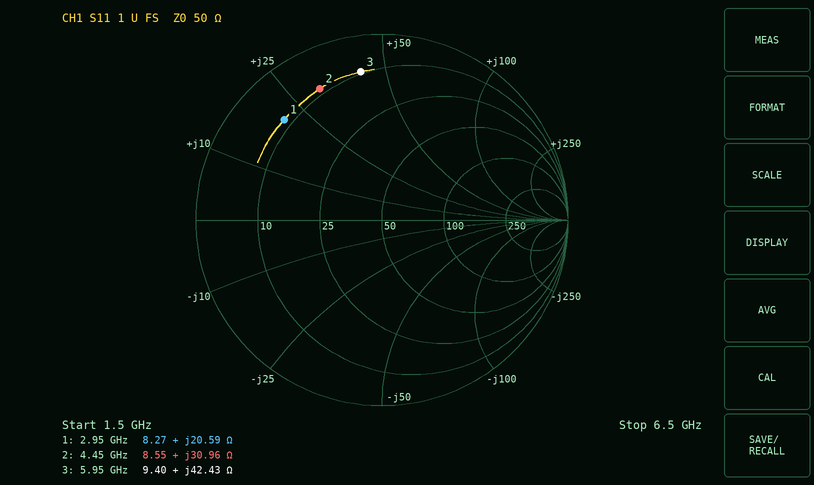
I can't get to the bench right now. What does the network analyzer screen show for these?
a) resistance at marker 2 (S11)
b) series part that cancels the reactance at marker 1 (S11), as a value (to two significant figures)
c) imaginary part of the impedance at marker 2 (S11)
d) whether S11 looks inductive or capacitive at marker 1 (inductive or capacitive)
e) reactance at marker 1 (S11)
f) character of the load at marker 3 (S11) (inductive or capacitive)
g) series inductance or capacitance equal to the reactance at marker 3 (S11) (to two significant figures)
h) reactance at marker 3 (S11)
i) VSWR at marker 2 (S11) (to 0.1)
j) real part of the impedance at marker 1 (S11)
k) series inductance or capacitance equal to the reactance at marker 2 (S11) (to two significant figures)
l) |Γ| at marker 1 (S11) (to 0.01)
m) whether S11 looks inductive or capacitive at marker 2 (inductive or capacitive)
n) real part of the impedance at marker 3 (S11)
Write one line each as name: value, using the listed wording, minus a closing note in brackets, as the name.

resistance at marker 2: 8.55 Ω
series part that cancels the reactance at marker 1 (S11), as a value: 2.6 pF
imaginary part of the impedance at marker 2: +30.96 Ω
whether S11 looks inductive or capacitive at marker 1: inductive
reactance at marker 1: +20.59 Ω
character of the load at marker 3 (S11): inductive
series inductance or capacitance equal to the reactance at marker 3 (S11): 1.1 nH
reactance at marker 3: +42.43 Ω
VSWR at marker 2 (S11): 8.1
real part of the impedance at marker 1: 8.27 Ω
series inductance or capacitance equal to the reactance at marker 2 (S11): 1.1 nH
|Γ| at marker 1 (S11): 0.75
whether S11 looks inductive or capacitive at marker 2: inductive
real part of the impedance at marker 3: 9.40 Ω
